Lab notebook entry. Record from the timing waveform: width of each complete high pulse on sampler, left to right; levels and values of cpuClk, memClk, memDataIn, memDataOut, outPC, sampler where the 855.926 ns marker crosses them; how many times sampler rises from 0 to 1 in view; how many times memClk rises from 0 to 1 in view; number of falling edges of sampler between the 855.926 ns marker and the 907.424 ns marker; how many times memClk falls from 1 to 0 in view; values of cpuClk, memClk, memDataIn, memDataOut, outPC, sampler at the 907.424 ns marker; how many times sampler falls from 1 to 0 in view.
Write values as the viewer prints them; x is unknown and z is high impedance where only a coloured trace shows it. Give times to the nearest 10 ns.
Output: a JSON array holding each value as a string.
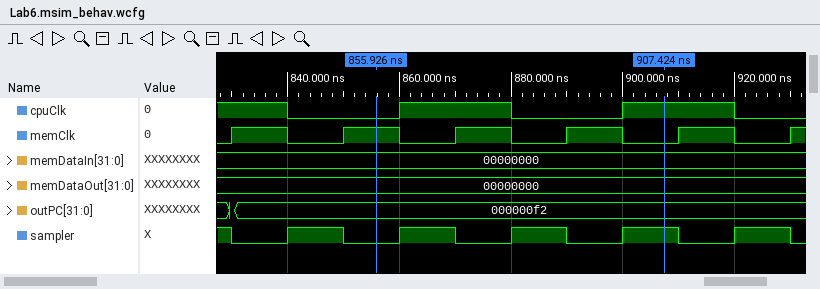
["10 ns, 10 ns, 10 ns, 10 ns, 10 ns", "cpuClk=0, memClk=1, memDataIn=00000000, memDataOut=00000000, outPC=000000f2, sampler=0", "5", "6", "2", "5", "cpuClk=1, memClk=0, memDataIn=00000000, memDataOut=00000000, outPC=000000f2, sampler=1", "6"]
